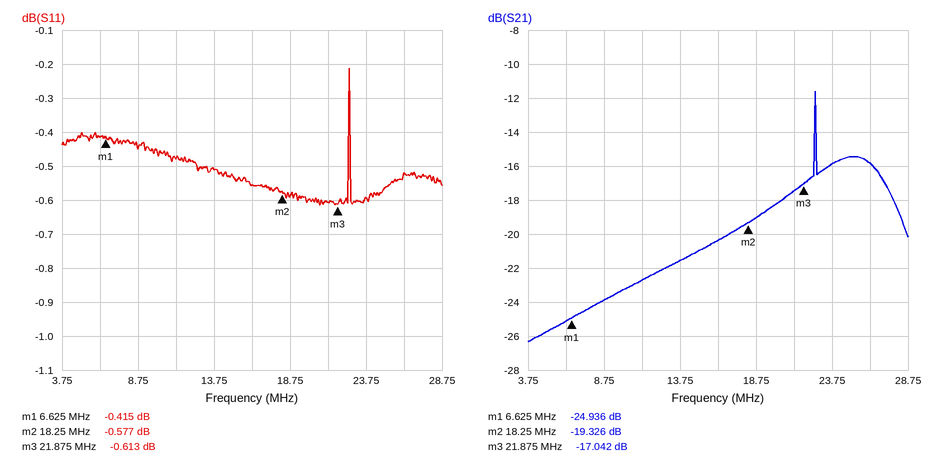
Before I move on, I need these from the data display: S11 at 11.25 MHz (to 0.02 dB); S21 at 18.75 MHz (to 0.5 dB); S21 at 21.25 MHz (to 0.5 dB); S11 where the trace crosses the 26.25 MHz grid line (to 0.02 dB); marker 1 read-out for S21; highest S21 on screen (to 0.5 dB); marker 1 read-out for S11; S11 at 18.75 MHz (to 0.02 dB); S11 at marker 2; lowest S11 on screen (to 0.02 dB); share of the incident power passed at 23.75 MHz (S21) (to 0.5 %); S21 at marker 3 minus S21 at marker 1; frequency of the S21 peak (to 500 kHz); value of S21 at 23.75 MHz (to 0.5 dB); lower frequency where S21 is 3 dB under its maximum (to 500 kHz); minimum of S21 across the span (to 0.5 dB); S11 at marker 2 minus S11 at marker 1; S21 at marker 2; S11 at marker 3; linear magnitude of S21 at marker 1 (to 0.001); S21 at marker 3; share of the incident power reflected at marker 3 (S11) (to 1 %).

-0.48 dB
-19.0 dB
-17.5 dB
-0.52 dB
-24.936 dB
-11.5 dB
-0.415 dB
-0.58 dB
-0.577 dB
-0.62 dB
2.5 %
7.894 dB
22.5 MHz
-16.0 dB
22.5 MHz
-26.5 dB
-0.162 dB
-19.326 dB
-0.613 dB
0.057
-17.042 dB
87 %
